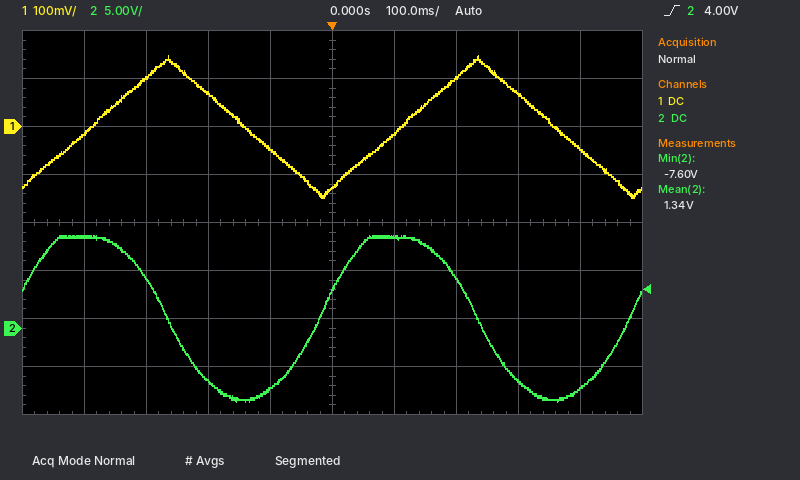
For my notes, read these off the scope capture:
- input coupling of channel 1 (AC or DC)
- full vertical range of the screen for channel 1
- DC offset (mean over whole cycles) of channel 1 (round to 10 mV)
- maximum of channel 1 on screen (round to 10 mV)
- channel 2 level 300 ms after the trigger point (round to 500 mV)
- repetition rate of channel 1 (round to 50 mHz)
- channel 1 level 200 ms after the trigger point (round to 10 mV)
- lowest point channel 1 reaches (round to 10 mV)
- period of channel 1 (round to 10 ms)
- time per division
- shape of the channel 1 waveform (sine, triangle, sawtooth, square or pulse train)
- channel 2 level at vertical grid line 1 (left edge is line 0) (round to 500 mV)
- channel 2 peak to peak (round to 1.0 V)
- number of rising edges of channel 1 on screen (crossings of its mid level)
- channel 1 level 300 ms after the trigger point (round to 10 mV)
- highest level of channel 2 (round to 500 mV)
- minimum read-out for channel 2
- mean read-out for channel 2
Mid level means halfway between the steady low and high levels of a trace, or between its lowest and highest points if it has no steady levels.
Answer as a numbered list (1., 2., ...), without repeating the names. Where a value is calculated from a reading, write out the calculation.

1. DC
2. 800 mV
3. (150 mV + (-150 mV)) / 2 ≈ 0 mV
4. 150 mV
5. -5.5 V
6. 1 / 500 ms ≈ 2.00 Hz
7. 100 mV
8. -150 mV
9. 500 ms
10. 100 ms
11. triangle
12. 9.5 V
13. 17.0 V
14. 2
15. 70 mV
16. 9.5 V
17. -7.60 V
18. 1.34 V
